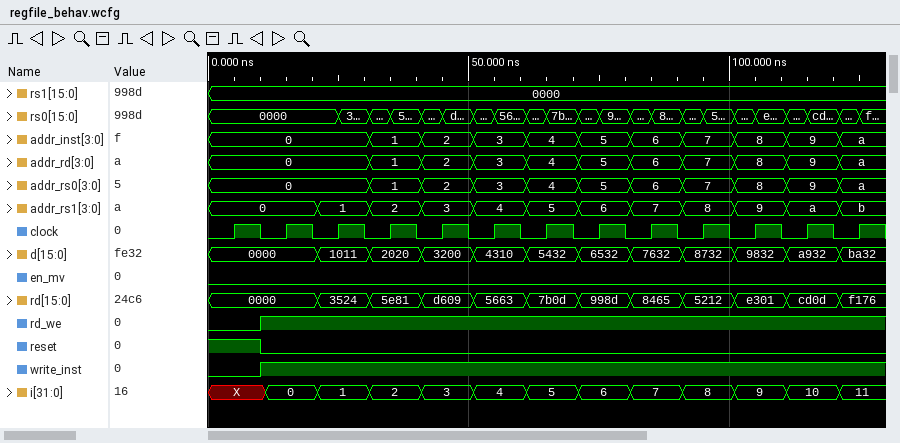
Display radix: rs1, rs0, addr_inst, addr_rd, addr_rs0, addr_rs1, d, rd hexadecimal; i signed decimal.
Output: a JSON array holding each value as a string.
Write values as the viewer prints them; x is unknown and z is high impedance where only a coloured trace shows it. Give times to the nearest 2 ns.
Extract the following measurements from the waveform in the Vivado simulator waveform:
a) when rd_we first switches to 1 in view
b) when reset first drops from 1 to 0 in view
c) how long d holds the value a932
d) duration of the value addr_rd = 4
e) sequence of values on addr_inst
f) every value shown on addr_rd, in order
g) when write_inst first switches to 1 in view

["10 ns", "10 ns", "10 ns", "10 ns", "0, 1, 2, 3, 4, 5, 6, 7, 8, 9, a", "0, 1, 2, 3, 4, 5, 6, 7, 8, 9, a", "10 ns"]
